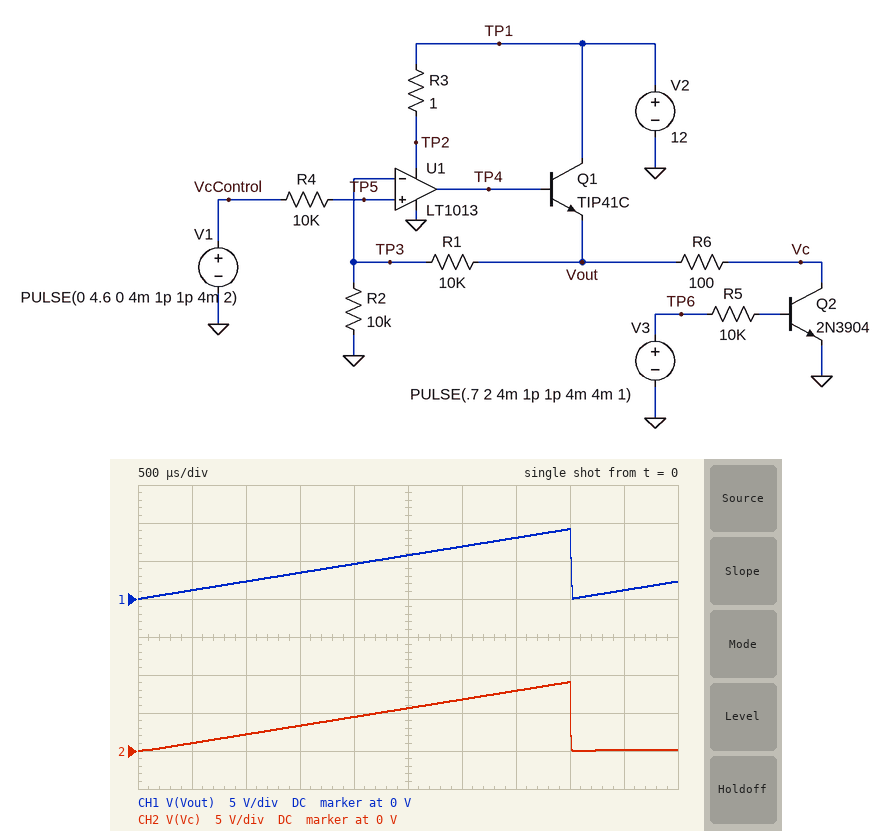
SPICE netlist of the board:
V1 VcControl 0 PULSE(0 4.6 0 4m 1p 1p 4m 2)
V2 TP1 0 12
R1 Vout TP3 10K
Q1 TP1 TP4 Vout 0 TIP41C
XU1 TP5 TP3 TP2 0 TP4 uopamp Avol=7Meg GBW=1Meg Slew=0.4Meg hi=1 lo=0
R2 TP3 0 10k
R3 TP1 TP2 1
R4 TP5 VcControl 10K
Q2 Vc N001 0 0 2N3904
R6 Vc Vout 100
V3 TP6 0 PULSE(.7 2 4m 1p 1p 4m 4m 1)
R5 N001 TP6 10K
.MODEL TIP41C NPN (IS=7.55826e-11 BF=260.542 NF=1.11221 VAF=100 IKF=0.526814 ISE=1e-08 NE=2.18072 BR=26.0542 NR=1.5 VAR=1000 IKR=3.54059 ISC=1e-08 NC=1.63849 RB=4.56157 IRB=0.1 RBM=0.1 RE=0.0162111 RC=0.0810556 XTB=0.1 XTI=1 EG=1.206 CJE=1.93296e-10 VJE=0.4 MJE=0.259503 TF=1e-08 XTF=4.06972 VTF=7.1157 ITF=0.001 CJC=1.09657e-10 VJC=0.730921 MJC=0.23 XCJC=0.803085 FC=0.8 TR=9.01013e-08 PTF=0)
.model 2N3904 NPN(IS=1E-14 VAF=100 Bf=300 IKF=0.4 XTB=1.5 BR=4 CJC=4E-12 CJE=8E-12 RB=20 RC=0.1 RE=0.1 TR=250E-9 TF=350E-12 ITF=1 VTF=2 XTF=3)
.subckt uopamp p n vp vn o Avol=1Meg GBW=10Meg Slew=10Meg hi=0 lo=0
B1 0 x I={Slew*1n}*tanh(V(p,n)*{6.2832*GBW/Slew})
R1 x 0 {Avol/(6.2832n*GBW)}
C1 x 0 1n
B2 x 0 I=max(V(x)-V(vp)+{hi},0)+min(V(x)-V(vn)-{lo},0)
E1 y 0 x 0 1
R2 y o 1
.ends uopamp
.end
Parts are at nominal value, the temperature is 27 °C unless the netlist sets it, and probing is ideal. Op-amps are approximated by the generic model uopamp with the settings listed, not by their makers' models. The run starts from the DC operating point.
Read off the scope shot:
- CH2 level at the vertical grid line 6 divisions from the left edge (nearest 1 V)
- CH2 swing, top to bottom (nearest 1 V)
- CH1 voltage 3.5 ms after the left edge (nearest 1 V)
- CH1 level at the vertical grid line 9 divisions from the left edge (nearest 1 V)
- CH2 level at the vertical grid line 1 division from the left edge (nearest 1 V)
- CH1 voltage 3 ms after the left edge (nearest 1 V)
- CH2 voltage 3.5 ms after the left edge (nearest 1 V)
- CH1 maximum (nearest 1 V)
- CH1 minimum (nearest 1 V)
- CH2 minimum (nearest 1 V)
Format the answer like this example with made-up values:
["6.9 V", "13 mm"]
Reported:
["7 V", "9 V", "8 V", "1 V", "1 V", "7 V", "8 V", "9 V", "0 V", "0 V"]
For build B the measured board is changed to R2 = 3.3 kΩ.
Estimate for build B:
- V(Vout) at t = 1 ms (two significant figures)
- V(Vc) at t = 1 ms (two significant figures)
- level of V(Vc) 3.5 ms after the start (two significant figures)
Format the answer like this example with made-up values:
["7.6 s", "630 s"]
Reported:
["4.6 V", "4.5 V", "10 V"]
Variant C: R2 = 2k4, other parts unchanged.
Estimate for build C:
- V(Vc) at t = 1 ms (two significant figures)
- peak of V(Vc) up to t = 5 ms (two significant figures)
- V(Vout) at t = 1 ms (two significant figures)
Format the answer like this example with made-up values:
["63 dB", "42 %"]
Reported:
["5.8 V", "10 V", "5.9 V"]
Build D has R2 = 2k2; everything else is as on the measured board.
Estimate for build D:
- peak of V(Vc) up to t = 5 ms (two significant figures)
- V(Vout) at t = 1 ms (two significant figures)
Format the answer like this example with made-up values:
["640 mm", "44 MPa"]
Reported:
["10 V", "6.4 V"]
